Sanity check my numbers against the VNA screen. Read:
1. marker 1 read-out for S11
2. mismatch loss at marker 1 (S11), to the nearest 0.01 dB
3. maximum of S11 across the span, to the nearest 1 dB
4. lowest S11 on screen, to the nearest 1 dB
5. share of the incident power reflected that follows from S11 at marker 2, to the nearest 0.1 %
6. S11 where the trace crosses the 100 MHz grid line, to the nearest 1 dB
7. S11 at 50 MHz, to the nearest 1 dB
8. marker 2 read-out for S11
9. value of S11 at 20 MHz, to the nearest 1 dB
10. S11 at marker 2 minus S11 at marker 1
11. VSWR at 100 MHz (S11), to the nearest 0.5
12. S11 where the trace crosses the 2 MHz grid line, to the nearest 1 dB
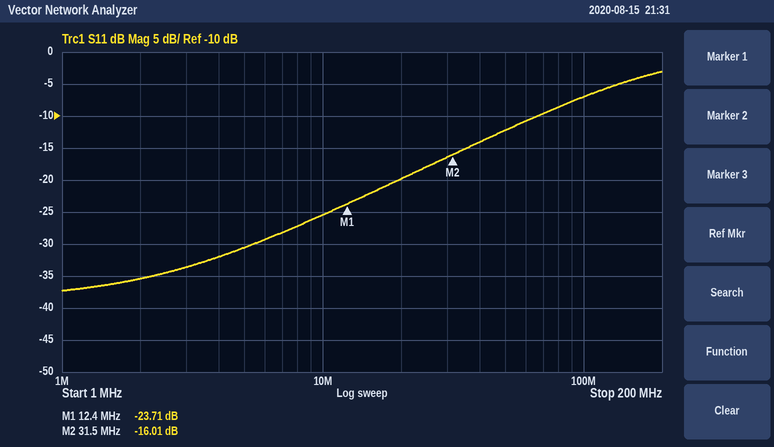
-23.71 dB
0.02 dB
-3 dB
-37 dB
2.5 %
-7 dB
-12 dB
-16.01 dB
-20 dB
7.70 dB
2.5
-35 dB
